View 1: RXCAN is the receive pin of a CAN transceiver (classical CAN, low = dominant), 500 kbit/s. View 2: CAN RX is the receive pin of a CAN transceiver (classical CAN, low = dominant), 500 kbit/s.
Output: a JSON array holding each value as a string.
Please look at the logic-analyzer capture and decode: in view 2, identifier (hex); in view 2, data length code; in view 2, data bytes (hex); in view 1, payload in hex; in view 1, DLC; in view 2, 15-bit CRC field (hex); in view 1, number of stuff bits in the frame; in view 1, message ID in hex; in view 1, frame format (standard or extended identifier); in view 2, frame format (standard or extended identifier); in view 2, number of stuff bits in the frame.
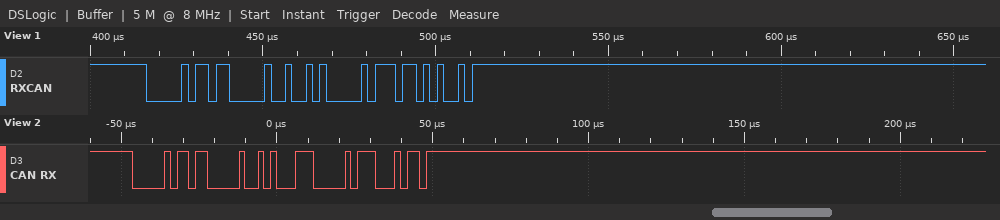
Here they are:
["0x036", "1", "47", "28", "1", "0x01C5", "3", "0x036", "standard", "standard", "3"]
